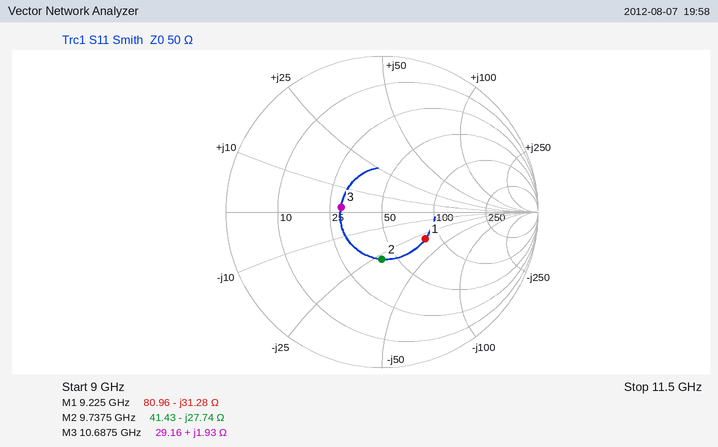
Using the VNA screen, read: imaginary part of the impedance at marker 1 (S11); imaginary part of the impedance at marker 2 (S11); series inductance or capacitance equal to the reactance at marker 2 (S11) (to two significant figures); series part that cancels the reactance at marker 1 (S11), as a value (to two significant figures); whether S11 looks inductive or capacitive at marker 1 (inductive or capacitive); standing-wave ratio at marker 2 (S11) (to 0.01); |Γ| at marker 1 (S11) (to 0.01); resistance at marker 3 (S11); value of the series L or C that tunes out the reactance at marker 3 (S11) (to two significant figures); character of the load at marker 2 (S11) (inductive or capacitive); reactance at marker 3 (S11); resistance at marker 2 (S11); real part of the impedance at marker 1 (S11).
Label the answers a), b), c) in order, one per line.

a) -31.28 Ω
b) -27.74 Ω
c) 590 fF
d) 540 pH
e) capacitive
f) 1.87
g) 0.33
h) 29.16 Ω
i) 7.7 pF
j) capacitive
k) +1.93 Ω
l) 41.43 Ω
m) 80.96 Ω
